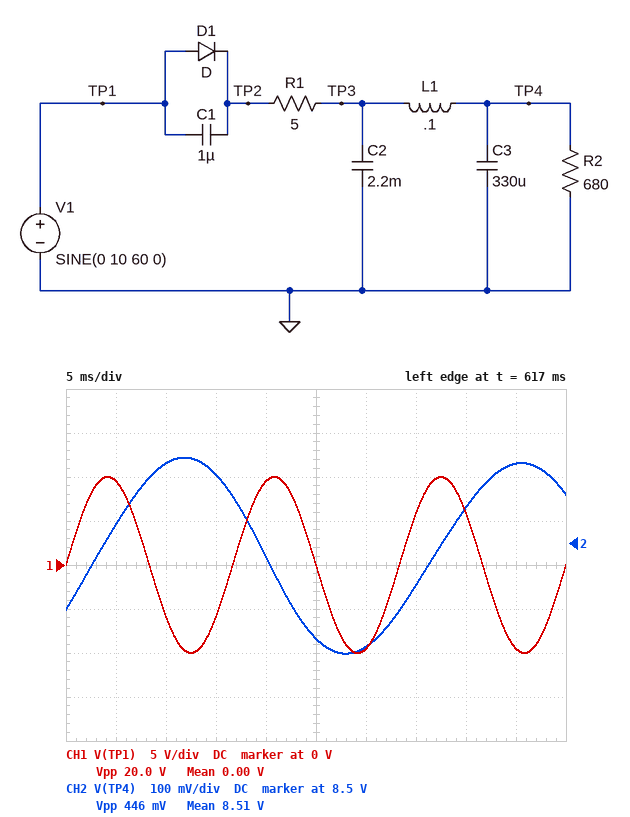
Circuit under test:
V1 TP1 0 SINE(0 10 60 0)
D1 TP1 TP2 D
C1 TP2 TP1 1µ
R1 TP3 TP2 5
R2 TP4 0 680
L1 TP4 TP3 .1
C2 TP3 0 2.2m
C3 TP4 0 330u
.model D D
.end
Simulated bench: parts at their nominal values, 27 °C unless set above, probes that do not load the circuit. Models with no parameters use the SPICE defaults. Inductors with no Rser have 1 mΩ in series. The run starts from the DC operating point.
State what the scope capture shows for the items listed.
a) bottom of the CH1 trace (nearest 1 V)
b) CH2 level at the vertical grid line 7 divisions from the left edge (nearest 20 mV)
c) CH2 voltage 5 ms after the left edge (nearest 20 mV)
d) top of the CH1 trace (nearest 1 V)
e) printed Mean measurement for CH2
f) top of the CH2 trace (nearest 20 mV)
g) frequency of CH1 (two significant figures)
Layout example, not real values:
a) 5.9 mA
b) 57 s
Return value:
a) -10 V
b) 8.40 V
c) 8.54 V
d) 10 V
e) 8.51 V
f) 8.70 V
g) 60 Hz
